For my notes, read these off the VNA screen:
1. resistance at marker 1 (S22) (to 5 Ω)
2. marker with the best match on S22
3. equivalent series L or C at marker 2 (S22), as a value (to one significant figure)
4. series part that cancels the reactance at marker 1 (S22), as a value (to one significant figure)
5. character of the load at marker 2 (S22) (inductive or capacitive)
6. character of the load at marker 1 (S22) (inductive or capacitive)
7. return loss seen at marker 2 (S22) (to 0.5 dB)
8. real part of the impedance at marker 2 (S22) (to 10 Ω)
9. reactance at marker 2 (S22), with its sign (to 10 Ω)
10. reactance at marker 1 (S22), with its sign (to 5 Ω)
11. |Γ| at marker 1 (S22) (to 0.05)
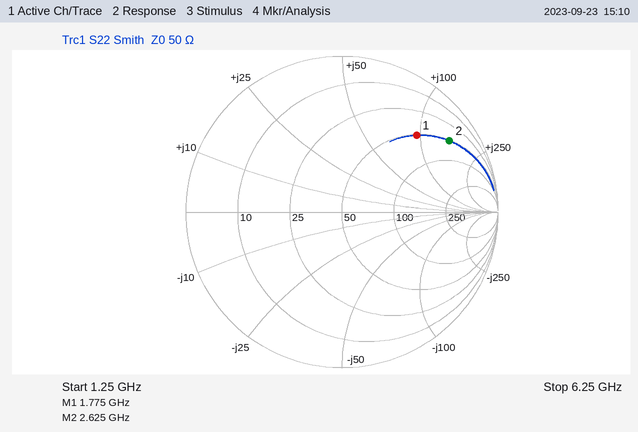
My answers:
50 Ω
marker 1
9 nH
900 fF
inductive
inductive
1.5 dB
50 Ω
+150 Ω
+95 Ω
0.70
